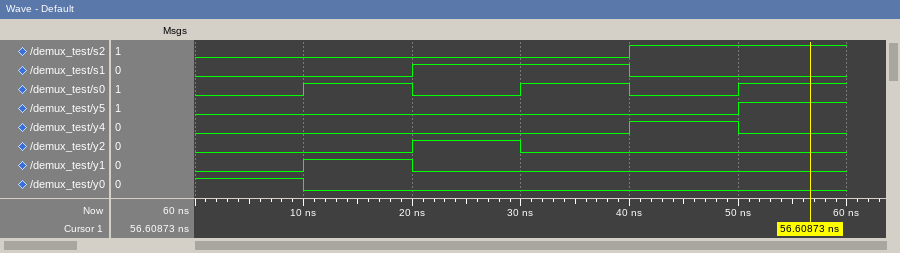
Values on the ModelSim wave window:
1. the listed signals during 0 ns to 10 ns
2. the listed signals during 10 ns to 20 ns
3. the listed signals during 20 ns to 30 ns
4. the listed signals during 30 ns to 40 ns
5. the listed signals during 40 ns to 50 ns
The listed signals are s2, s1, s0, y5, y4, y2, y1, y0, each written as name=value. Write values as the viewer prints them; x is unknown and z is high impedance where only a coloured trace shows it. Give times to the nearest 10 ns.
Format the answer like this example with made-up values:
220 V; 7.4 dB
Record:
s2=0, s1=0, s0=0, y5=0, y4=0, y2=0, y1=0, y0=1; s2=0, s1=0, s0=1, y5=0, y4=0, y2=0, y1=1, y0=0; s2=0, s1=1, s0=0, y5=0, y4=0, y2=1, y1=0, y0=0; s2=0, s1=1, s0=1, y5=0, y4=0, y2=0, y1=0, y0=0; s2=1, s1=0, s0=0, y5=0, y4=1, y2=0, y1=0, y0=0
